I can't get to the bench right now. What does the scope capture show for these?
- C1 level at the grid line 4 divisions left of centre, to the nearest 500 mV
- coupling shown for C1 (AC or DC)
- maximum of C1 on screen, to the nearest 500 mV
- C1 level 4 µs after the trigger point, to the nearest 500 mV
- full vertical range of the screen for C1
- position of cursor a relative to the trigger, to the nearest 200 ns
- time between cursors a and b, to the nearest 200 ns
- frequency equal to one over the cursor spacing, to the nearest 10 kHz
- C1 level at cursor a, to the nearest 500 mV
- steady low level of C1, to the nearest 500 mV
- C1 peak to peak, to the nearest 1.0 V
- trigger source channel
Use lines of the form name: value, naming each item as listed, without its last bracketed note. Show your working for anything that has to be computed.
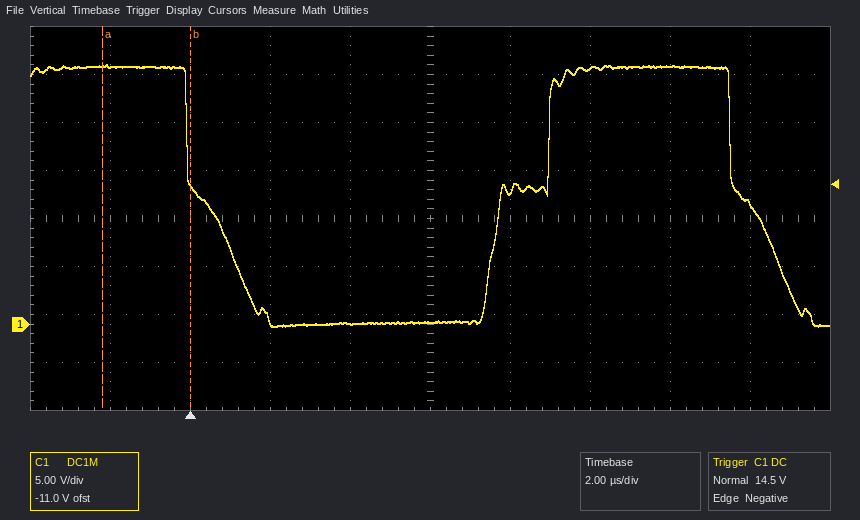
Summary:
C1 level at the grid line 4 divisions left of centre, to the nearest 500 mV: 27.0 V
coupling shown for C1: DC
maximum of C1 on screen, to the nearest 500 mV: 27.0 V
C1 level 4 µs after the trigger point, to the nearest 500 mV: 0.0 V
full vertical range of the screen for C1: 40 V
position of cursor a relative to the trigger, to the nearest 200 ns: -2.2 µs
time between cursors a and b, to the nearest 200 ns: 2.2 µs
frequency equal to one over the cursor spacing, to the nearest 10 kHz: 1 / 2.2 µs ≈ 450 kHz
C1 level at cursor a, to the nearest 500 mV: 27.0 V
steady low level of C1, to the nearest 500 mV: 0.0 V
C1 peak to peak, to the nearest 1.0 V: 27.0 V
trigger source channel: C1
